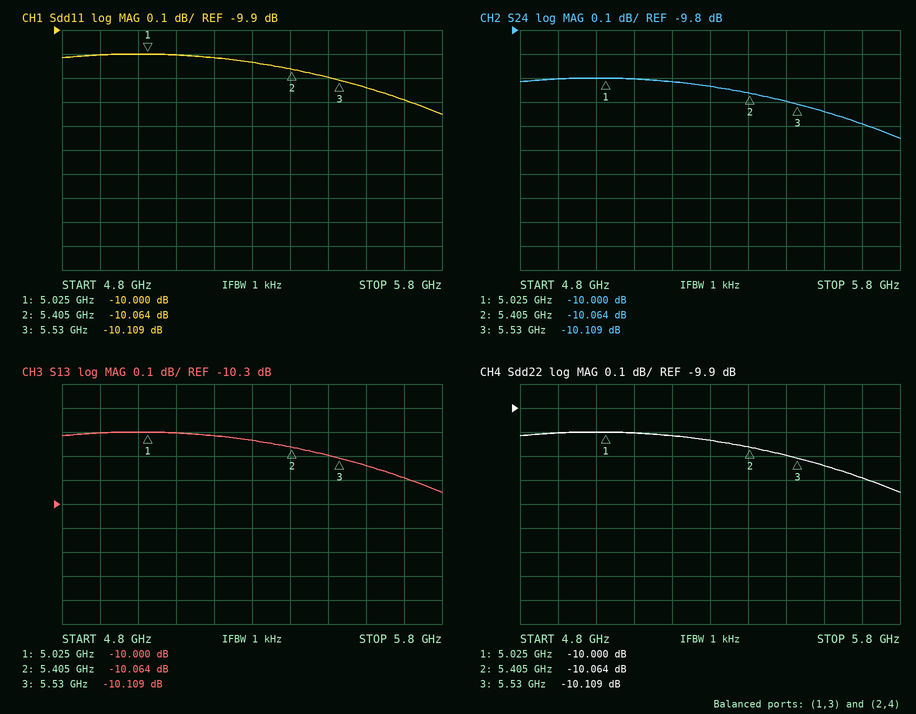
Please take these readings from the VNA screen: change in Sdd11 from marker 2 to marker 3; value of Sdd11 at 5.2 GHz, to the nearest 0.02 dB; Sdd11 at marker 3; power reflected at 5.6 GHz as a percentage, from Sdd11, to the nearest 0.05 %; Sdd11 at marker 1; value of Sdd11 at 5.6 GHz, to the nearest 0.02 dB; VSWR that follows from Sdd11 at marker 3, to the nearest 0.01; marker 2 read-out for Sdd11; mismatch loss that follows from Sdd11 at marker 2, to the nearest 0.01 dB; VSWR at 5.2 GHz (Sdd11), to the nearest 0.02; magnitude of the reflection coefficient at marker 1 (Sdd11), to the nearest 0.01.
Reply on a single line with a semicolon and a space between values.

-0.045 dB; -10.02 dB; -10.109 dB; 9.70 %; -10.000 dB; -10.14 dB; 1.91; -10.064 dB; 0.45 dB; 1.92; 0.32
